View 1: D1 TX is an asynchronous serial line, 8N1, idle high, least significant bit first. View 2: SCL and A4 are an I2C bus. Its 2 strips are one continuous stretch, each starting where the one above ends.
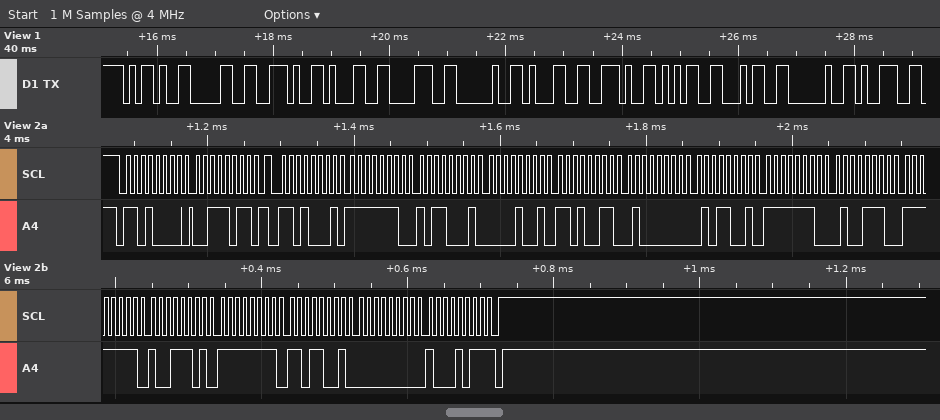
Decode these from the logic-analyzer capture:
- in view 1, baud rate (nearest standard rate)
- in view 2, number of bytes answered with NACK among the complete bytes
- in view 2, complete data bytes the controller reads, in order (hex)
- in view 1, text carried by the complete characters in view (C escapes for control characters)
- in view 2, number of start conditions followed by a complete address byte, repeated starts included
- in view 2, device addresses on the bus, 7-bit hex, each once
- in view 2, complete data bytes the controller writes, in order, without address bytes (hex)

9600 baud
1
FE B1 09 D3 40 59 FE 4E FF 9D FF D9 00 8B
"-0.18 1.54 9"
2
0x68
3B
